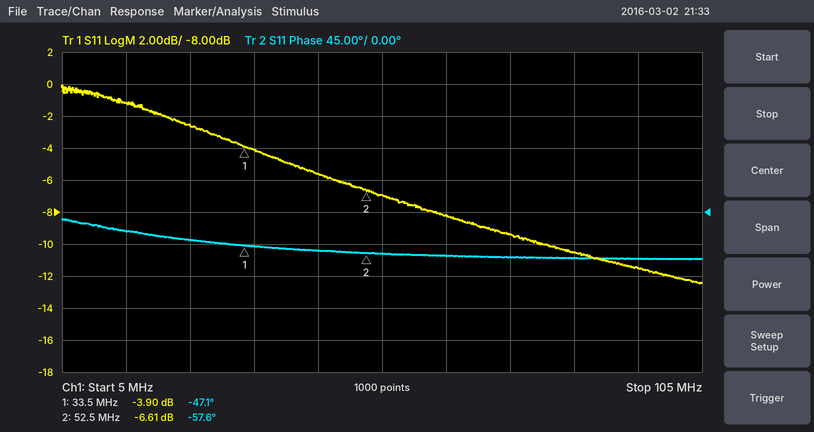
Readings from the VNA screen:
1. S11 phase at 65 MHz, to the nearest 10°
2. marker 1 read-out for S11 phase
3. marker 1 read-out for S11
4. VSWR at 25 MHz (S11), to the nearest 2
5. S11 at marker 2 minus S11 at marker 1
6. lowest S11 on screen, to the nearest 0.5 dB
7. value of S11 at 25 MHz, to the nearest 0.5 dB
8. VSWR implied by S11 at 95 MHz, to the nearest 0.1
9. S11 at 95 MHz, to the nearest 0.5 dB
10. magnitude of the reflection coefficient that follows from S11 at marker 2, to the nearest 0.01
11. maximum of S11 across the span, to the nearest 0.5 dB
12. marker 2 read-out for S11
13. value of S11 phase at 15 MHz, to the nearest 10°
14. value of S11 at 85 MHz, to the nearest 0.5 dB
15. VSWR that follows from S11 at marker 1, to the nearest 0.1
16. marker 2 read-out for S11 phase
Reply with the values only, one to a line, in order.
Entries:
-60°
-47.1°
-3.90 dB
6
-2.71 dB
-12.5 dB
-2.5 dB
1.7
-11.5 dB
0.47
0.0 dB
-6.61 dB
-30°
-10.5 dB
4.5
-57.6°
